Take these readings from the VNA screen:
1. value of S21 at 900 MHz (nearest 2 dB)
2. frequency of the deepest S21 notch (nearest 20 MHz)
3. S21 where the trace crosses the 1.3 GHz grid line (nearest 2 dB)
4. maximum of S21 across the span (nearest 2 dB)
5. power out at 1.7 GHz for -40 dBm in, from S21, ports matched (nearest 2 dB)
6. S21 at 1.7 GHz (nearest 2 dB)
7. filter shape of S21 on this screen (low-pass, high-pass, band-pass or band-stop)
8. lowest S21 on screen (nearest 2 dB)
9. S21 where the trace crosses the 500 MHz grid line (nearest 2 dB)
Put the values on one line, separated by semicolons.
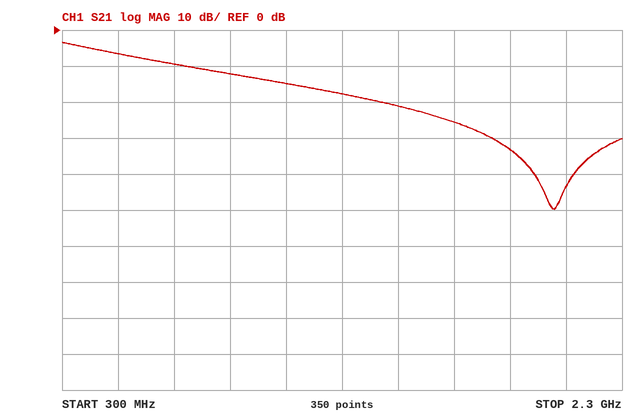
-12 dB; 2.06 GHz; -18 dB; -4 dB; -66 dBm; -26 dB; low-pass; -50 dB; -6 dB
